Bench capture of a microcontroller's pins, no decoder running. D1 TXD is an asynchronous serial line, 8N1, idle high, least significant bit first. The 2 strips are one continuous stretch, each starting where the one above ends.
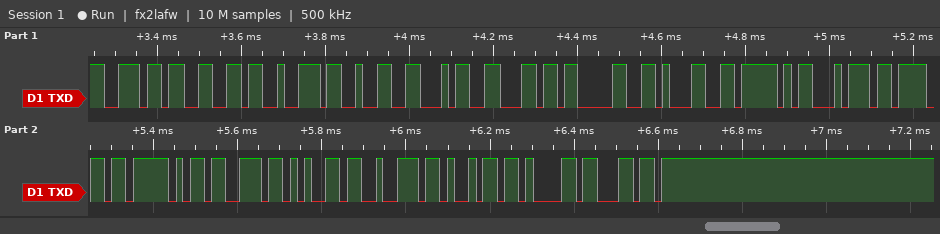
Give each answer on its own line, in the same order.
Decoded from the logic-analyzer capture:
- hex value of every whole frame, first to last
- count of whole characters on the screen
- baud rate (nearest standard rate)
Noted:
6E 66 72 32 34 6C 30 31 5F 74 6F 5F 73 65 72 69 61 6C
18
57600 baud
